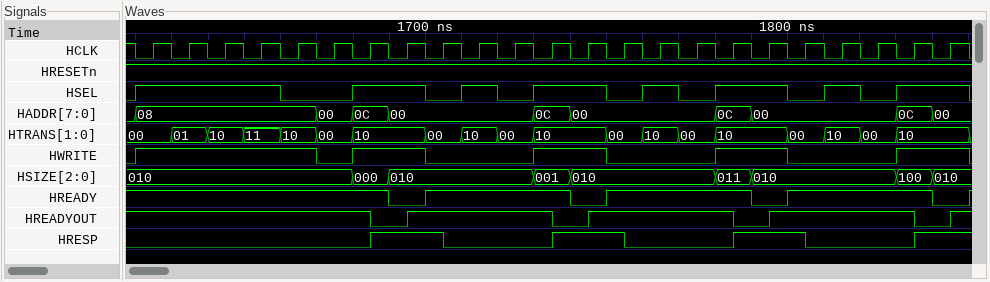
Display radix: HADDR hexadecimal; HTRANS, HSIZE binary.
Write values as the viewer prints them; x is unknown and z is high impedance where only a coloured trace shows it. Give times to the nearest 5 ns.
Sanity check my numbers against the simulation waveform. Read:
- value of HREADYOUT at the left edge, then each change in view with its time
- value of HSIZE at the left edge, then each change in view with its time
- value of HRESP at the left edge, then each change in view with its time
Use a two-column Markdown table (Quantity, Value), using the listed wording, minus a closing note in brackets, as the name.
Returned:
| Quantity | Value |
|---|---|
| value of HREADYOUT at the left edge, then each change in view with its time | 1, 0 at 1685 ns, 1 at 1695 ns, 0 at 1735 ns, 1 at 1745 ns, 0 at 1785 ns, 1 at 1795 ns, 0 at 1835 ns, 1 at 1845 ns |
| value of HSIZE at the left edge, then each change in view with its time | 010, 000 at 1680 ns, 010 at 1690 ns, 001 at 1730 ns, 010 at 1740 ns, 011 at 1780 ns, 010 at 1790 ns, 100 at 1830 ns, 010 at 1840 ns |
| value of HRESP at the left edge, then each change in view with its time | 0, 1 at 1685 ns, 0 at 1705 ns, 1 at 1735 ns, 0 at 1755 ns, 1 at 1785 ns, 0 at 1805 ns, 1 at 1835 ns |
